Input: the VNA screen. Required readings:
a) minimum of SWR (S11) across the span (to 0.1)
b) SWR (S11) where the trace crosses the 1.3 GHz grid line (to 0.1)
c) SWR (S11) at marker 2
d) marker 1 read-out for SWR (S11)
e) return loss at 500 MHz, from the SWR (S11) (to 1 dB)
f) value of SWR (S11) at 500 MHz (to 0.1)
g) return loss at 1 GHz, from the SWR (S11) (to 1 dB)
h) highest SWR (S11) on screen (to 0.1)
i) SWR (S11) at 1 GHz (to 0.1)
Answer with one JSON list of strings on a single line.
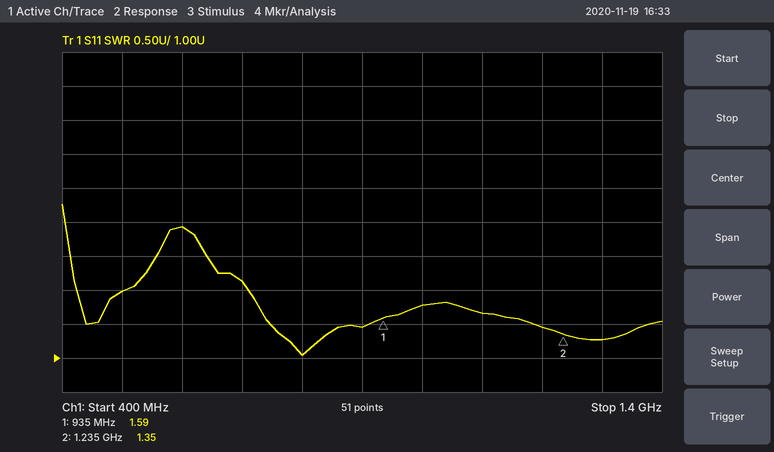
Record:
["1.0", "1.3", "1.35", "1.59", "10 dB", "2.0", "11 dB", "3.3", "1.8"]
